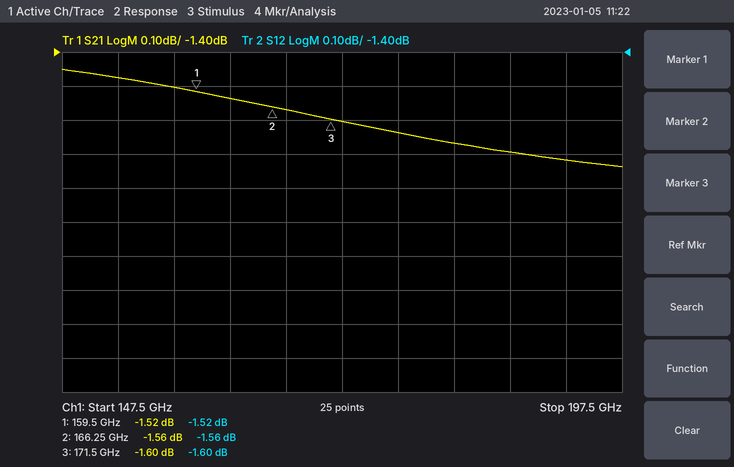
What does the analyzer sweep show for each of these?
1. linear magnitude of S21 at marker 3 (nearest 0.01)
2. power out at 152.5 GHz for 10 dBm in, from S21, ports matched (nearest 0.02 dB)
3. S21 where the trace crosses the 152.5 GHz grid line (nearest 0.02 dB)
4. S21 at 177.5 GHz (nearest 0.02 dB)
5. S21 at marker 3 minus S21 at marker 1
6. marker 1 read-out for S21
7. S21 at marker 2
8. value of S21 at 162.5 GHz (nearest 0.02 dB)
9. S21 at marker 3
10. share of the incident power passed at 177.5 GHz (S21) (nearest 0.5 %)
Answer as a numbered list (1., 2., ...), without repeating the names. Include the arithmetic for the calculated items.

1. 10^(-1.6/20) ≈ 0.83
2. 10 dBm + (-1.48 dB) = 8.52 dBm
3. -1.48 dB
4. -1.64 dB
5. -1.6 − (-1.52) = -0.08 dB
6. -1.52 dB
7. -1.56 dB
8. -1.54 dB
9. -1.60 dB
10. 10^(-1.64/10) ≈ 68.5 %
